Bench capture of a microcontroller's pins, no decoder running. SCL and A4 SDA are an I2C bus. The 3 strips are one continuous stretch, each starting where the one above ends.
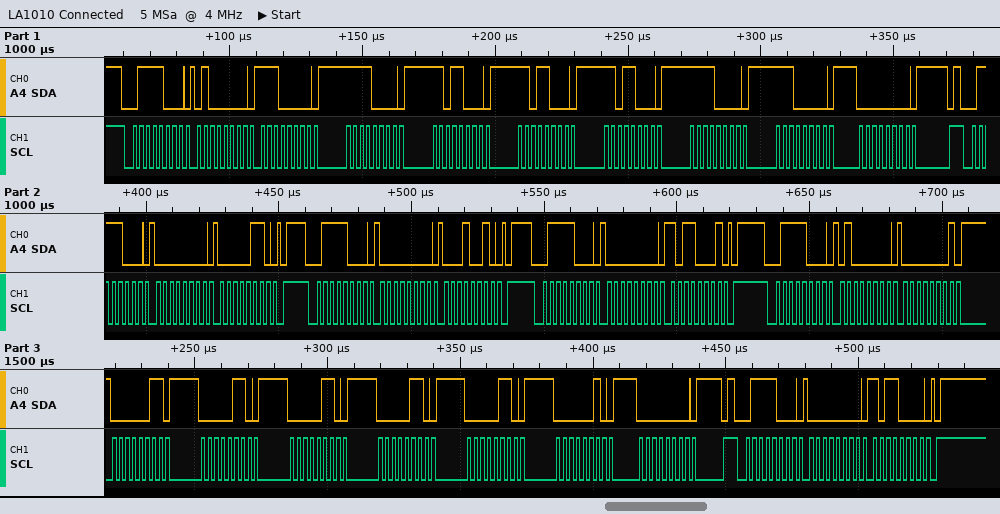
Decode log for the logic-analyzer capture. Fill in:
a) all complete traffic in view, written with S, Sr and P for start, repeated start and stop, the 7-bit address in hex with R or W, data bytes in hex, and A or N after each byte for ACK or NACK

S 3CW A 40 A E0 A F0 A D8 A D8 A D8 A F0 A E0 A 00 A P S 3CW A 00 A 06 A P S 3CW A 00 A 12 A P S 3CW A 00 A B1 A P S 3CW A 40 A 01 A 03 A 06 A 06 A 06 A 06 A 02 A 00 A P S 3CW A 00 A B0 A P
